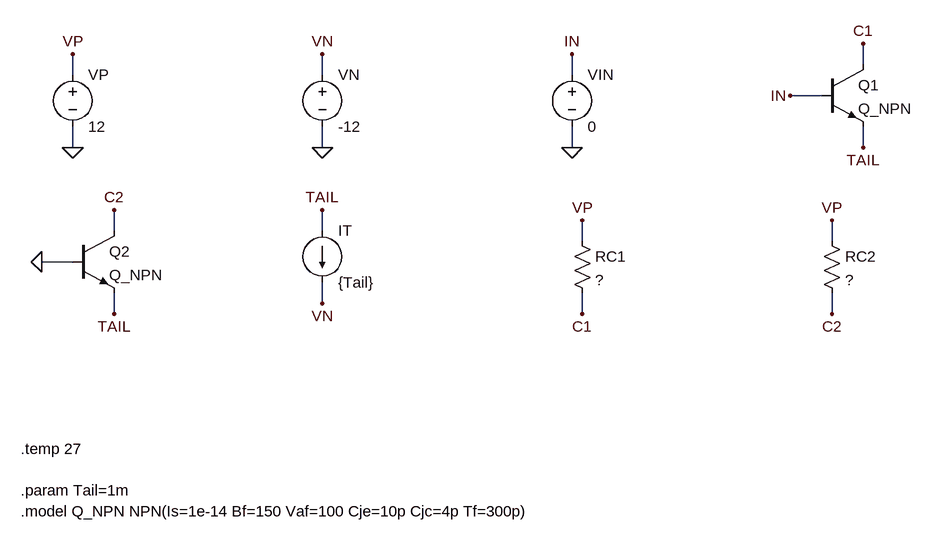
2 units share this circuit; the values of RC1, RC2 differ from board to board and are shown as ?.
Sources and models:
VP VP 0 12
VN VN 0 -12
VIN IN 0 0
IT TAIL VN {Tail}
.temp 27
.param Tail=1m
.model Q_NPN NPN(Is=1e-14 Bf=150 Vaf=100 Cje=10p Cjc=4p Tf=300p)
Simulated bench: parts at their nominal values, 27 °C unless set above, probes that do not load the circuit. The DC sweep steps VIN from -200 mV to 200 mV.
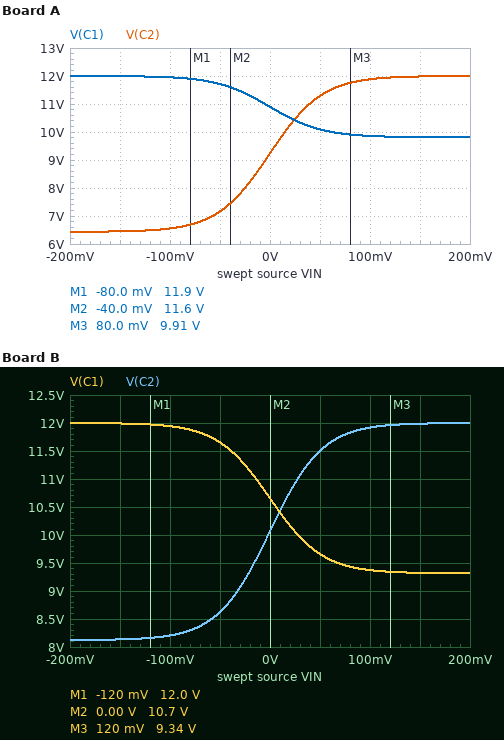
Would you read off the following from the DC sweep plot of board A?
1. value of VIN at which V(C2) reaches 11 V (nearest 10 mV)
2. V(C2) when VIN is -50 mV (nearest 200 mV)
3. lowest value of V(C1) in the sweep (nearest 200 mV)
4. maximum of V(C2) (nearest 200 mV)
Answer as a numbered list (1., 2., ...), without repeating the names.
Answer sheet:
1. 40 mV
2. 7.2 V
3. 9.8 V
4. 12.0 V
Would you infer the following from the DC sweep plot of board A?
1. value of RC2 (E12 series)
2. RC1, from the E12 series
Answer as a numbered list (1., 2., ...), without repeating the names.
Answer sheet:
1. 5.6 kΩ
2. 2.2 kΩ
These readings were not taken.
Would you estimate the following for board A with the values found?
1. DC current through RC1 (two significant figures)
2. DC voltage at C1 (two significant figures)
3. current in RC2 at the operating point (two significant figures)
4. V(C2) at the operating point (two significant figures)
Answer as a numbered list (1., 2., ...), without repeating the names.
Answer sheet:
1. 500 µA
2. 11 V
3. 490 µA
4. 9.2 V
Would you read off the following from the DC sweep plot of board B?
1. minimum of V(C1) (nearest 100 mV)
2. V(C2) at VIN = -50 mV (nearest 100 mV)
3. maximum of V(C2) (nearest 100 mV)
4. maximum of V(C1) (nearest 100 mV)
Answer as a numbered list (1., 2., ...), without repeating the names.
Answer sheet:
1. 9.3 V
2. 8.6 V
3. 12.0 V
4. 12.0 V
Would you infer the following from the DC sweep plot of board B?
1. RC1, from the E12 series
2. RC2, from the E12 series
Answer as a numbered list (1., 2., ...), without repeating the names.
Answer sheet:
1. 2.7 kΩ
2. 3.9 kΩ
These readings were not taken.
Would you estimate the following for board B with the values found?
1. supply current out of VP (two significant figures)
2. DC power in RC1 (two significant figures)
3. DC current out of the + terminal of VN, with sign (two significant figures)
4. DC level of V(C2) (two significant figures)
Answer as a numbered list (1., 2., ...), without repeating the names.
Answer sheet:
1. 990 µA
2. 670 µW
3. -1.0 mA
4. 10 V
